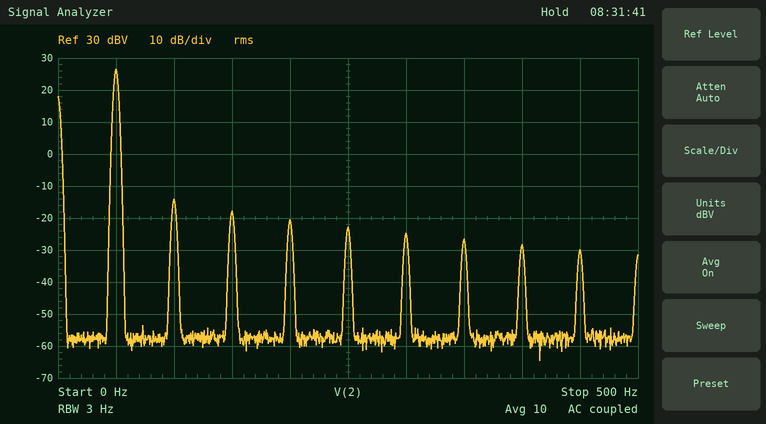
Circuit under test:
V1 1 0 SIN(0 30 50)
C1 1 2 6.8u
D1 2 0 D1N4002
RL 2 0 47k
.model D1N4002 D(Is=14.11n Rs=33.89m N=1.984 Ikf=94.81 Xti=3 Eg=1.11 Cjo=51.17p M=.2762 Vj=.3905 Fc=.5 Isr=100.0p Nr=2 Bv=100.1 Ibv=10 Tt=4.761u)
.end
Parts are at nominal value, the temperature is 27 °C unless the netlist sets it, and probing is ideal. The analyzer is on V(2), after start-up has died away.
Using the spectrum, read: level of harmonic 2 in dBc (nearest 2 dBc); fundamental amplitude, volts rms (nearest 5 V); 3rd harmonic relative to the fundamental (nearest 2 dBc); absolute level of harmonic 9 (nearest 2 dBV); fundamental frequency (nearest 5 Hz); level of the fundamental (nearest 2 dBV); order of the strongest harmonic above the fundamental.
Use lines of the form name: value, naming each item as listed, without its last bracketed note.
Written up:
level of harmonic 2 in dBc: -40 dBc
fundamental amplitude, volts rms: 20 V
3rd harmonic relative to the fundamental: -44 dBc
absolute level of harmonic 9: -30 dBV
fundamental frequency: 50 Hz
level of the fundamental: 26 dBV
order of the strongest harmonic above the fundamental: 2
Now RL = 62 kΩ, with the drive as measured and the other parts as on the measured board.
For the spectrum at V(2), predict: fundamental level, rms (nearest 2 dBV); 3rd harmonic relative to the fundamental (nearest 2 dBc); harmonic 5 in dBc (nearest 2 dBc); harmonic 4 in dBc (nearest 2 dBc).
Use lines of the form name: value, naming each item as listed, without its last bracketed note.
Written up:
fundamental level, rms: 26 dBV
3rd harmonic relative to the fundamental: -46 dBc
harmonic 5 in dBc: -52 dBc
harmonic 4 in dBc: -50 dBc
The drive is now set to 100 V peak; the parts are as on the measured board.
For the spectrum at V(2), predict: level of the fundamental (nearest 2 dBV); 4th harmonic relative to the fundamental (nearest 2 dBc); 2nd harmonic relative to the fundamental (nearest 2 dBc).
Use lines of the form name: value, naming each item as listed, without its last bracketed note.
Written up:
level of the fundamental: 32 dBV
4th harmonic relative to the fundamental: -54 dBc
2nd harmonic relative to the fundamental: -46 dBc
